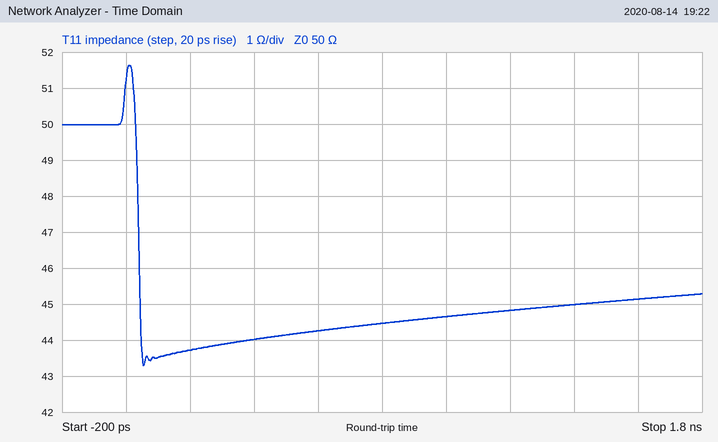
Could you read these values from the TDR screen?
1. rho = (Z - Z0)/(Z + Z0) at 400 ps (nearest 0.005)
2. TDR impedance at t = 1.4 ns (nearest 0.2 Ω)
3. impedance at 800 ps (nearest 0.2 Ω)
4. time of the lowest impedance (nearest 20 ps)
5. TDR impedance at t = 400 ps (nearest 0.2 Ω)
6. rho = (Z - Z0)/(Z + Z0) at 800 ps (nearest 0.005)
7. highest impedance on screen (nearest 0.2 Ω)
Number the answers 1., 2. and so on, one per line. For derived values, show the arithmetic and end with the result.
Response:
1. (44 − 50)/(44 + 50) ≈ -0.0638, so -0.065 to the nearest 0.005
2. 45.0 Ω
3. 44.4 Ω
4. 60 ps
5. 44.0 Ω
6. (44.4 − 50)/(44.4 + 50) ≈ -0.0593, so -0.060 to the nearest 0.005
7. 51.6 Ω
